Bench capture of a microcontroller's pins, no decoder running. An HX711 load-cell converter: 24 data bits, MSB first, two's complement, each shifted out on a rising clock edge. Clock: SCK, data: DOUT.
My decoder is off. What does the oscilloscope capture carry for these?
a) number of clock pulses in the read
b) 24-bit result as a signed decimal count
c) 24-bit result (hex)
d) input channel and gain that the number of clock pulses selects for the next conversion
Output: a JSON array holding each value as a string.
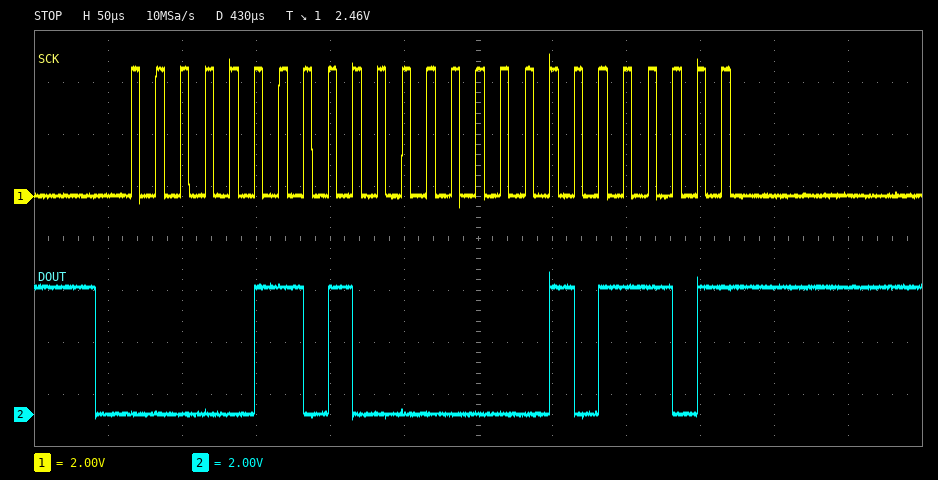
["25", "426077", "0x06805D", "channel A, gain 128"]
